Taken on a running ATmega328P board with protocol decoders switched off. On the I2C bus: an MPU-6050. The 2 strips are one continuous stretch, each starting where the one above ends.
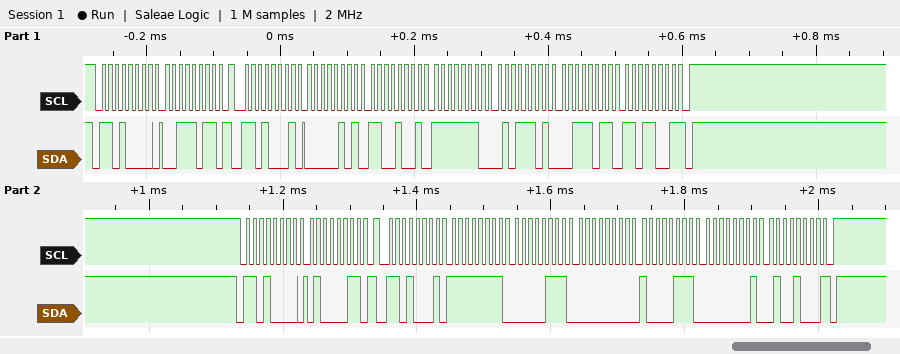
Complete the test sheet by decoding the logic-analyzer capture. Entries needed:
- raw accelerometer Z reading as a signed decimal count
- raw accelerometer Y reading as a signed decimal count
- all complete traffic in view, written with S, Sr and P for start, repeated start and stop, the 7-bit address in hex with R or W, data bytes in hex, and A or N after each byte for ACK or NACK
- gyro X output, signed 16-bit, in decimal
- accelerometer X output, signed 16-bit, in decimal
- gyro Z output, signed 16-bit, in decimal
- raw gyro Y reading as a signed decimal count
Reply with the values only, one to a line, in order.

15321
-419
S 68W A 3B A Sr 68R A 05 A C9 A FE A 5D A 3B A D9 N P S 68W A 43 A Sr 68R A FF A 07 A 00 A 87 A 01 A 48 N P
-249
1481
328
135
